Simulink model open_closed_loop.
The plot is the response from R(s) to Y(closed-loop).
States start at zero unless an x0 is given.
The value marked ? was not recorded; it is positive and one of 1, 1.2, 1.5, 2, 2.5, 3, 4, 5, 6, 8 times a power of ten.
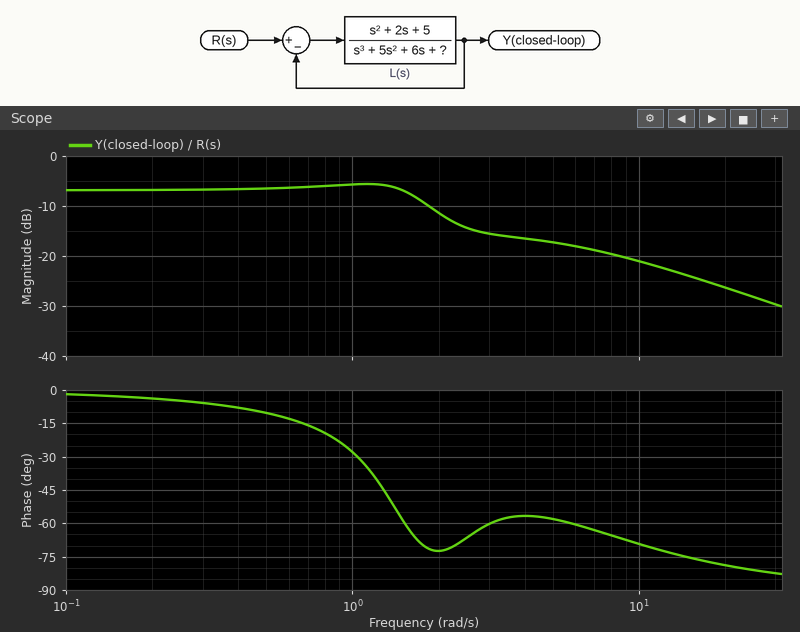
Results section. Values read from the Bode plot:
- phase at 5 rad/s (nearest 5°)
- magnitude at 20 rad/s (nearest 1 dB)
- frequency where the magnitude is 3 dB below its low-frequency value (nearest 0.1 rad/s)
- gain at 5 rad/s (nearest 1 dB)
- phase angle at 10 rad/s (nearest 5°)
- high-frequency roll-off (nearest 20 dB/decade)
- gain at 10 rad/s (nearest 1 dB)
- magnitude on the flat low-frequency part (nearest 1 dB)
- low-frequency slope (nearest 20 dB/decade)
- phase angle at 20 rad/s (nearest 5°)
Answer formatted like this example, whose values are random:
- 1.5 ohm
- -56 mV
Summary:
- -60°
- -26 dB
- 1.8 rad/s
- -17 dB
- -70°
- -20 dB/decade
- -21 dB
- -7 dB
- 0 dB/decade
- -80°
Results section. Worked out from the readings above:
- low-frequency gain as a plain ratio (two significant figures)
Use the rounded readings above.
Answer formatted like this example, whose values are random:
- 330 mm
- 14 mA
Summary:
- 0.45
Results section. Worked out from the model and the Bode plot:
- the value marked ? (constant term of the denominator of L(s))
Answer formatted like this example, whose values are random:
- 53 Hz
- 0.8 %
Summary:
- 6
